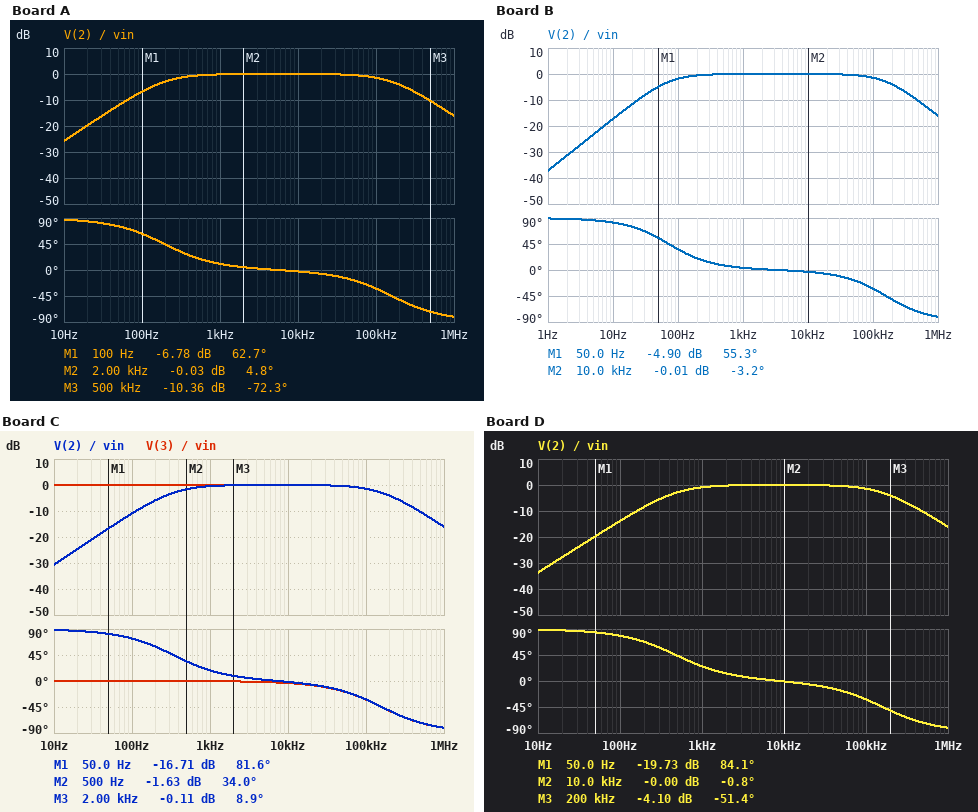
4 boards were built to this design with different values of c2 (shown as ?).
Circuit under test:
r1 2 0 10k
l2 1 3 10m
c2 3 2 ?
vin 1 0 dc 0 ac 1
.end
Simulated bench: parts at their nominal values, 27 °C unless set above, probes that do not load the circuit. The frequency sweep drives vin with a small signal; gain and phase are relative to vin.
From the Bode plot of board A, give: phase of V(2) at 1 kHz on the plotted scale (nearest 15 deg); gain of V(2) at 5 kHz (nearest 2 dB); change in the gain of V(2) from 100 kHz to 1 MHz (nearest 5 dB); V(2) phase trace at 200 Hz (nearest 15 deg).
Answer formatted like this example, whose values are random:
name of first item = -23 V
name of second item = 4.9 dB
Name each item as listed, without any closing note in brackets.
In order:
phase of V(2) at 1 kHz on the plotted scale = 15 deg
gain of V(2) at 5 kHz = 0 dB
change in the gain of V(2) from 100 kHz to 1 MHz = -15 dB
V(2) phase trace at 200 Hz = 45 deg
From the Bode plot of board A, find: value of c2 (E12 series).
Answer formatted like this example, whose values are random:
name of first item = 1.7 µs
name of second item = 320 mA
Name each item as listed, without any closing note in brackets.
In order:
value of c2 = 82 nF
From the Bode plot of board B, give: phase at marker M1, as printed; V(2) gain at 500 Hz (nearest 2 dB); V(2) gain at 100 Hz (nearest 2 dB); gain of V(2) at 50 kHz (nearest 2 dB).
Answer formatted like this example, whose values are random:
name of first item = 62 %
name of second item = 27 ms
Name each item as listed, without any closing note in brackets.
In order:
phase at marker M1, as printed = 55.3 deg
V(2) gain at 500 Hz = 0 dB
V(2) gain at 100 Hz = -2 dB
gain of V(2) at 50 kHz = 0 dB
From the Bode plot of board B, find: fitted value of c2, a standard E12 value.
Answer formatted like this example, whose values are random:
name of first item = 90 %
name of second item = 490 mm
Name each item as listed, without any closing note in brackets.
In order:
fitted value of c2, a standard E12 value = 220 nF
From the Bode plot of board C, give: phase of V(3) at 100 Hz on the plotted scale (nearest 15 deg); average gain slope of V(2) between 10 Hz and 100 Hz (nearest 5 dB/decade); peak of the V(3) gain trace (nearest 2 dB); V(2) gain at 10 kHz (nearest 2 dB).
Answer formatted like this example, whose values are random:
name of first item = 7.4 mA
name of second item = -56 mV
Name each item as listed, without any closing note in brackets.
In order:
phase of V(3) at 100 Hz on the plotted scale = 0 deg
average gain slope of V(2) between 10 Hz and 100 Hz = 20 dB/decade
peak of the V(3) gain trace = 0 dB
V(2) gain at 10 kHz = 0 dB
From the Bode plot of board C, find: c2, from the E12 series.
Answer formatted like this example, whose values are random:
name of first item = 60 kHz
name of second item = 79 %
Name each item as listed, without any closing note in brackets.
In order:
c2, from the E12 series = 47 nF
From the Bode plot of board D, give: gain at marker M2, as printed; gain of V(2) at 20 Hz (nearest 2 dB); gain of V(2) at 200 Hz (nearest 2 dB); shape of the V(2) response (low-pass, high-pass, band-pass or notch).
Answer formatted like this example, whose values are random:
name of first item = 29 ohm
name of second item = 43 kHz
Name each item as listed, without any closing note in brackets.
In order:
gain at marker M2, as printed = -0.00 dB
gain of V(2) at 20 Hz = -28 dB
gain of V(2) at 200 Hz = -8 dB
shape of the V(2) response = band-pass
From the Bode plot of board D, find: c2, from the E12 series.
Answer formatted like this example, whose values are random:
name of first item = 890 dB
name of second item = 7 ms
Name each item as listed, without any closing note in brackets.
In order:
c2, from the E12 series = 33 nF
